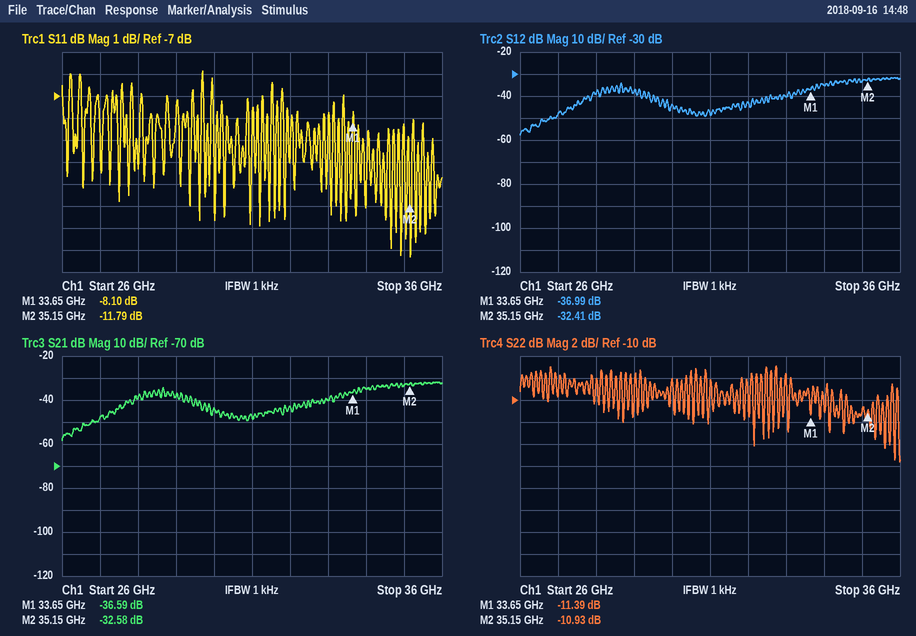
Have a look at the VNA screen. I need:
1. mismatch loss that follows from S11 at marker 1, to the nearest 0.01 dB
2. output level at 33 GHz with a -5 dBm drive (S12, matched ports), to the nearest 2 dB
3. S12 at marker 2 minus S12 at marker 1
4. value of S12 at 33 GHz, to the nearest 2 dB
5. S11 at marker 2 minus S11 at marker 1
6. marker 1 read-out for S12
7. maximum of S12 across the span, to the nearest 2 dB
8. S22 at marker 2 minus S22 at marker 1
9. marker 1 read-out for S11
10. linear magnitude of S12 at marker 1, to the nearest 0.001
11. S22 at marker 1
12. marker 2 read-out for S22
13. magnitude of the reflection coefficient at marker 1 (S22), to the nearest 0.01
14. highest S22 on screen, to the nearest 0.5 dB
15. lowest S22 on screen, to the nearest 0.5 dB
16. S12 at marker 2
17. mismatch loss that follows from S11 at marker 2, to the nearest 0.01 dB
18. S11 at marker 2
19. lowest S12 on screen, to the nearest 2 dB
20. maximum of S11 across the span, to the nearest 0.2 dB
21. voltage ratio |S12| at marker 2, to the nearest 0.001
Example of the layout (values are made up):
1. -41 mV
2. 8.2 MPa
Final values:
1. 0.73 dB
2. -46 dBm
3. 4.58 dB
4. -40 dB
5. -3.69 dB
6. -36.99 dB
7. -32 dB
8. 0.46 dB
9. -8.10 dB
10. 0.014
11. -11.39 dB
12. -10.93 dB
13. 0.27
14. -7.0 dB
15. -15.5 dB
16. -32.41 dB
17. 0.30 dB
18. -11.79 dB
19. -58 dB
20. -5.8 dB
21. 0.024
